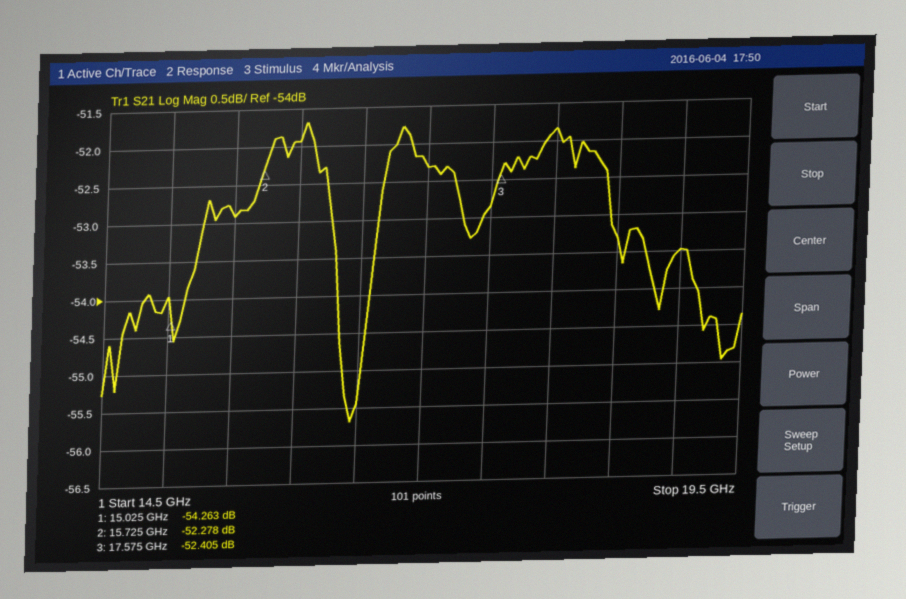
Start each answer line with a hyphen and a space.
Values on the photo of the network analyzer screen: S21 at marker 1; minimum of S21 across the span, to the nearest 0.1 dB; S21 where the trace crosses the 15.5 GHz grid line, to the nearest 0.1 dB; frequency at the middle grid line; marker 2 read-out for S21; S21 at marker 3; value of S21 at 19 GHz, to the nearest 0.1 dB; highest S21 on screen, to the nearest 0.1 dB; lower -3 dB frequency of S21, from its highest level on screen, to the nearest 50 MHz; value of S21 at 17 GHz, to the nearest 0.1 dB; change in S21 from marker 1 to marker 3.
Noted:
- -54.263 dB
- -55.7 dB
- -52.9 dB
- 17 GHz
- -52.278 dB
- -52.405 dB
- -53.5 dB
- -51.7 dB
- 14.65 GHz
- -52.3 dB
- 1.858 dB
